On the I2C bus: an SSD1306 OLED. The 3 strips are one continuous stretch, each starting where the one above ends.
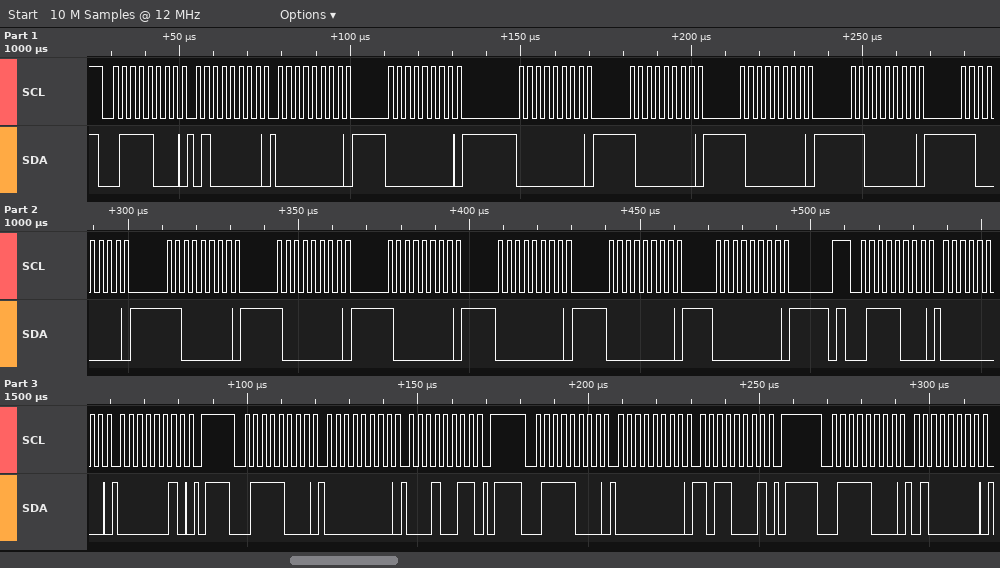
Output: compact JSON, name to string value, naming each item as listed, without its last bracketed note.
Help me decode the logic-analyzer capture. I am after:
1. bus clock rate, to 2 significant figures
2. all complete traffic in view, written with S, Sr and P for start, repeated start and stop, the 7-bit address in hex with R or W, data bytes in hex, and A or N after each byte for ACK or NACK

{"bus clock rate, to 2 significant figures": "400 kHz", "all complete traffic in view, written with S, Sr and P for start, repeated start and stop, the 7-bit address in hex with R or W, data bytes in hex, and A or N after each byte for ACK or NACK": "S 3CW A 40 A 00 A 00 A 00 A 80 A 80 A C0 A C0 A C0 A 80 A 80 A 00 A 00 A 00 A P S 3CW A 00 A 02 A P S 3CW A 00 A 13 A P S 3CW A 00 A B1 A P S 3CW A 40 A"}
